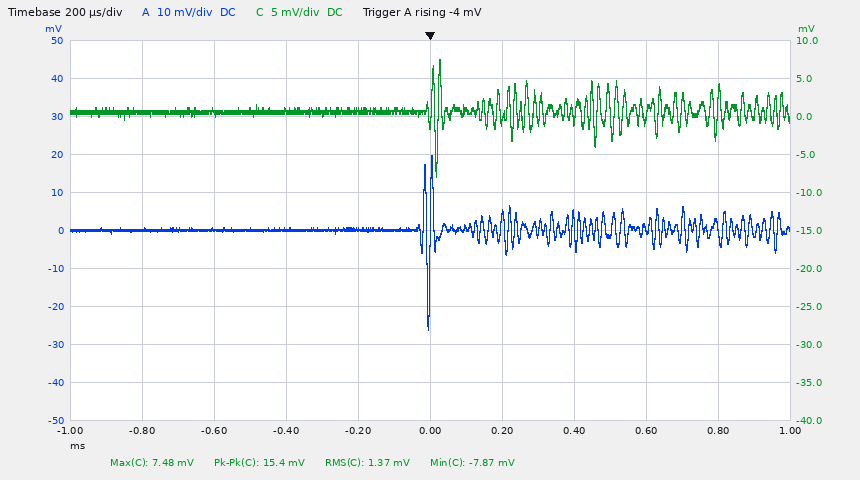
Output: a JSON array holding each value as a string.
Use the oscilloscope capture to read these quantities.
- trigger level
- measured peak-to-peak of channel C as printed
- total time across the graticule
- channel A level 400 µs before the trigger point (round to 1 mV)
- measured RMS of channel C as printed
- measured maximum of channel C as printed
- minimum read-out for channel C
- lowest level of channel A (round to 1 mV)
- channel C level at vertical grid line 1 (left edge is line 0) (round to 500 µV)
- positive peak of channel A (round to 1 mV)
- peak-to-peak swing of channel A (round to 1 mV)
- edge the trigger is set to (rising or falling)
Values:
["-4 mV", "15.4 mV", "2 ms", "0 mV", "1.37 mV", "7.48 mV", "-7.87 mV", "-26 mV", "500 µV", "20 mV", "46 mV", "rising"]
